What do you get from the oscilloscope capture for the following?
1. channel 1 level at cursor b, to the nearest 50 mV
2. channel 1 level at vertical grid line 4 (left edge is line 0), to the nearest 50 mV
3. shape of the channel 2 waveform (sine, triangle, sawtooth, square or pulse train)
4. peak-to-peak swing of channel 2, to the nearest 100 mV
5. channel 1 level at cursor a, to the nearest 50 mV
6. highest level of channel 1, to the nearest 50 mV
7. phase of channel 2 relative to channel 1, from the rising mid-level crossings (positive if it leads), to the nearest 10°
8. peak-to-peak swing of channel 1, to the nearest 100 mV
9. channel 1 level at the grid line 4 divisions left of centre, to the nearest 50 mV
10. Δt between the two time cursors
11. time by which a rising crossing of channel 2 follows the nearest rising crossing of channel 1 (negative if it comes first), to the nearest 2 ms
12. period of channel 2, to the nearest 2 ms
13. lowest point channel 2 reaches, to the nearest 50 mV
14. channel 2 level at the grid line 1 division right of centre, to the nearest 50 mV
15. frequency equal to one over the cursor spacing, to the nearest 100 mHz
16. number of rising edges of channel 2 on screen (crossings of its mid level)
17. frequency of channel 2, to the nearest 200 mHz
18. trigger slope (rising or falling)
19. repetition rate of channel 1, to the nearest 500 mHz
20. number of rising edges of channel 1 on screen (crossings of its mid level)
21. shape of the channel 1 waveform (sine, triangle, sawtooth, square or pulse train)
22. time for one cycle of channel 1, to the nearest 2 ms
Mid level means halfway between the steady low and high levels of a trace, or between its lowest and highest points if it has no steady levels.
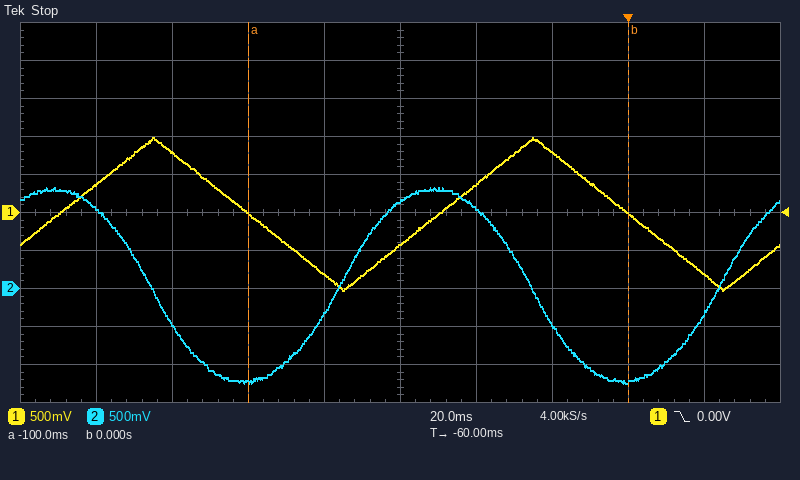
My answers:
0 mV
-800 mV
sine
2.60 V
0 mV
1.00 V
+90°
2.00 V
350 mV
100 ms
-26 ms
100 ms
-1.25 V
1.05 V
10.0 Hz
2
10.0 Hz
falling
10.0 Hz
2
triangle
100 ms
